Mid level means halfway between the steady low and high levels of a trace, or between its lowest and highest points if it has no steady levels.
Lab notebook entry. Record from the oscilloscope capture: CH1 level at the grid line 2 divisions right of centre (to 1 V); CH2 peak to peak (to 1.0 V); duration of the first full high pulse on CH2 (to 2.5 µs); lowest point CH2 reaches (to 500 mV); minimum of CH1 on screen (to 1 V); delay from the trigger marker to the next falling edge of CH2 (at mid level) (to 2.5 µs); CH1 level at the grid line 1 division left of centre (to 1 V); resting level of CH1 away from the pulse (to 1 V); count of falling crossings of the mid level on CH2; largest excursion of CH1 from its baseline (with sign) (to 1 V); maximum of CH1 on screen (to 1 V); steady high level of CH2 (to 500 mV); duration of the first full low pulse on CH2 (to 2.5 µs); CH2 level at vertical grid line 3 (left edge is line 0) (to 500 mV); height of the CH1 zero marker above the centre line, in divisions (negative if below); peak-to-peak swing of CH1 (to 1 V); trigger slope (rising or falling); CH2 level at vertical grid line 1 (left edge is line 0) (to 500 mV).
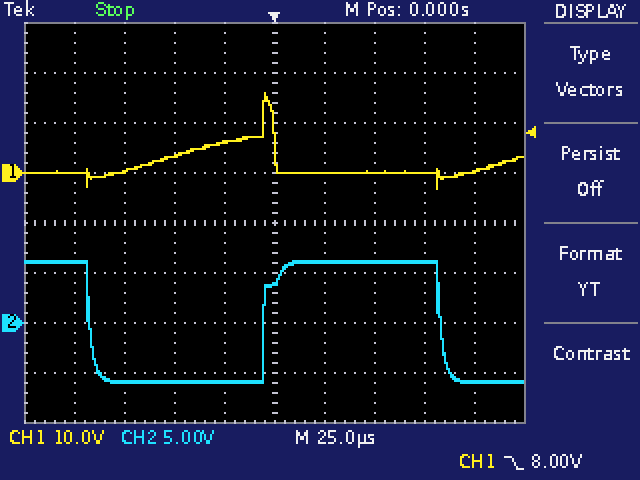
0 V
12.0 V
87.5 µs
-6.0 V
-3 V
82.5 µs
6 V
0 V
2
+16 V
16 V
6.0 V
87.5 µs
-6.0 V
+1.0 div
19 V
falling
6.0 V
